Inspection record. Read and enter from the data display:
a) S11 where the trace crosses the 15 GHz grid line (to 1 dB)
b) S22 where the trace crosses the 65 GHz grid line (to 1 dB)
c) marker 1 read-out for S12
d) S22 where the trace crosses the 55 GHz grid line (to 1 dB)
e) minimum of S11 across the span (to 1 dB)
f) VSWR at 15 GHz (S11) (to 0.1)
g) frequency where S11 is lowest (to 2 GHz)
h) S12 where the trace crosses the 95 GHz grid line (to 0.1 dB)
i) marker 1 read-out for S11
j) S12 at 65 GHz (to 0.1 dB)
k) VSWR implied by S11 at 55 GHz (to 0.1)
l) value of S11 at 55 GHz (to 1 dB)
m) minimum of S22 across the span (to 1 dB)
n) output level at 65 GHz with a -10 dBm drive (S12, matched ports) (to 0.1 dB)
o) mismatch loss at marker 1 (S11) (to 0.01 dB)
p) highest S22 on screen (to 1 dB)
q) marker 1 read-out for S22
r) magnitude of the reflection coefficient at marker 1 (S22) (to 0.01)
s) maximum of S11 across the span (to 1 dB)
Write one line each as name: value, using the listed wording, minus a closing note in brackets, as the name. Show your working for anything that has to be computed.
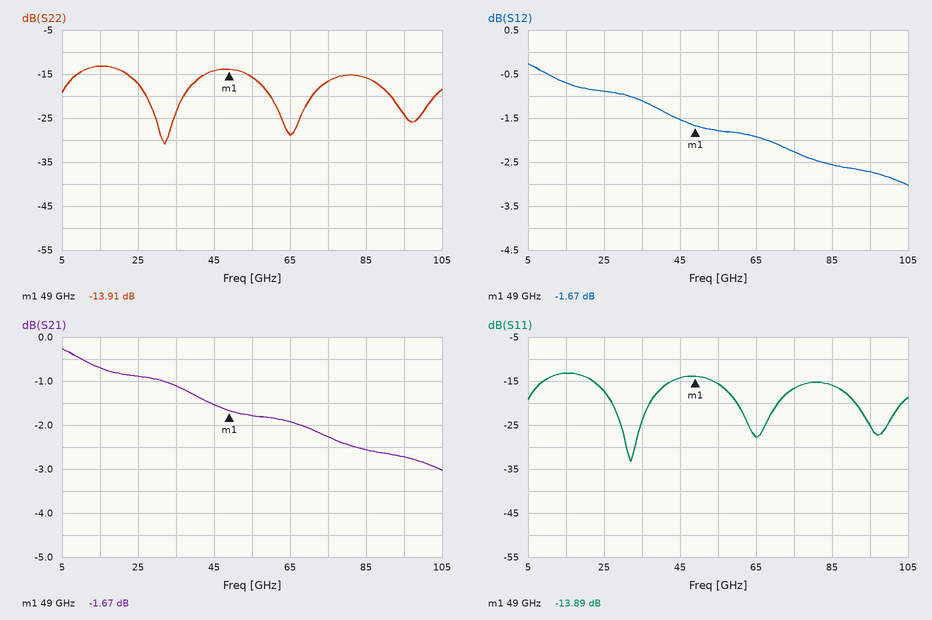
S11 where the trace crosses the 15 GHz grid line: -13 dB
S22 where the trace crosses the 65 GHz grid line: -29 dB
marker 1 read-out for S12: -1.67 dB
S22 where the trace crosses the 55 GHz grid line: -16 dB
minimum of S11 across the span: -33 dB
VSWR at 15 GHz (S11): |Γ| = 10^(-13/20) = 0.2239; VSWR = (1 + 0.2239)/(1 − 0.2239) ≈ 1.6
frequency where S11 is lowest: 32 GHz
S12 where the trace crosses the 95 GHz grid line: -2.7 dB
marker 1 read-out for S11: -13.89 dB
S12 at 65 GHz: -1.9 dB
VSWR implied by S11 at 55 GHz: |Γ| = 10^(-16/20) = 0.1585; VSWR = (1 + 0.1585)/(1 − 0.1585) ≈ 1.4
value of S11 at 55 GHz: -16 dB
minimum of S22 across the span: -31 dB
output level at 65 GHz with a -10 dBm drive (S12, matched ports): -10 dBm + (-1.9 dB) = -11.9 dBm
mismatch loss at marker 1 (S11): −10 log10(1 − 10^(-13.89/10)) ≈ 0.18 dB
highest S22 on screen: -13 dB
marker 1 read-out for S22: -13.91 dB
magnitude of the reflection coefficient at marker 1 (S22): 10^(-13.91/20) ≈ 0.20
maximum of S11 across the span: -13 dB
